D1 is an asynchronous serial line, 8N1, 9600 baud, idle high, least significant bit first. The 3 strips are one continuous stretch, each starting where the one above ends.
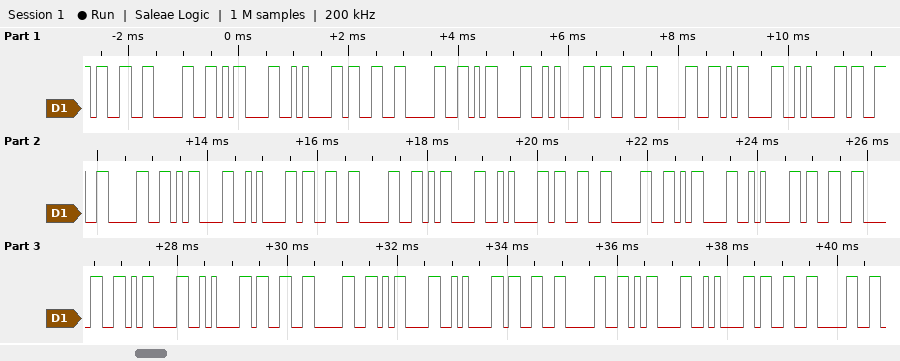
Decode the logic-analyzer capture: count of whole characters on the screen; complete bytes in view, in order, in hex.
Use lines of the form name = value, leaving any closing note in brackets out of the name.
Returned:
count of whole characters on the screen = 38
complete bytes in view, in order, in hex = 0x33 0x30 0x0D 0x0A 0x33 0x30 0x0D 0x0A 0x33 0x30 0x0D 0x0A 0x33 0x30 0x0D 0x0A 0x33 0x30 0x0D 0x0A 0x33 0x30 0x0D 0x0A 0x33 0x30 0x0D 0x0A 0x33 0x30 0x0D 0x0A 0x33 0x30 0x0D 0x0A 0x33 0x30
